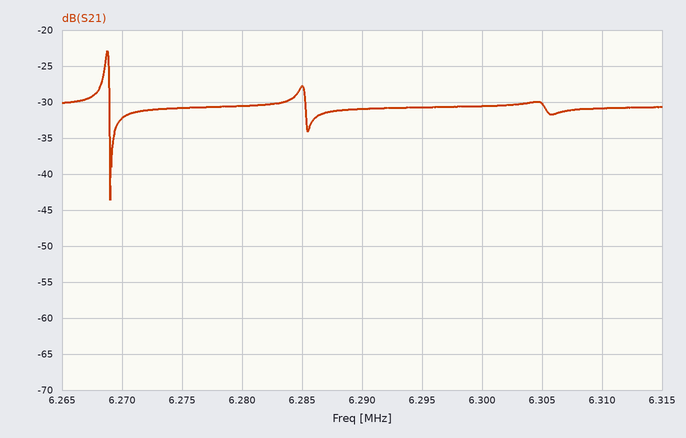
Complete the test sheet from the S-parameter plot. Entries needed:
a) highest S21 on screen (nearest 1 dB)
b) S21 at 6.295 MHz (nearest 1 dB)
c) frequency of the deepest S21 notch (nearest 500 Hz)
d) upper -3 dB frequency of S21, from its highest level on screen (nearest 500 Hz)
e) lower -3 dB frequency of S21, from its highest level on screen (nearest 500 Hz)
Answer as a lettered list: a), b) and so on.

a) -23 dB
b) -31 dB
c) 6.2690 MHz
d) 6.2690 MHz
e) 6.2685 MHz
